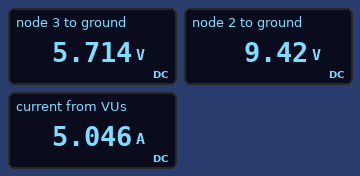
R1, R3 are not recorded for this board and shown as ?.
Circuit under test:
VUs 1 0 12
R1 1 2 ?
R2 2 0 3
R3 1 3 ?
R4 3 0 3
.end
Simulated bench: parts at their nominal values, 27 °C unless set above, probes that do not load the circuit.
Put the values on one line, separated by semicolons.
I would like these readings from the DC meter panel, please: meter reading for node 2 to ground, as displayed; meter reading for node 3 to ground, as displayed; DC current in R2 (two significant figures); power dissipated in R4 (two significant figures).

9.42 V; 5.714 V; 3.1 A; 11 W
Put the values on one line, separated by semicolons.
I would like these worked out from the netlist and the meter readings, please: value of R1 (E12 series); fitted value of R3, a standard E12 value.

0.82 Ω; 3.3 Ω
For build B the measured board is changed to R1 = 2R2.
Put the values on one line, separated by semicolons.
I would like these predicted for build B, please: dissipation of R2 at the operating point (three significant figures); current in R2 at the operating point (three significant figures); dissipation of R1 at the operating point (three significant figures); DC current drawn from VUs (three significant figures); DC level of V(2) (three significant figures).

16.0 W; 2.31 A; 11.7 W; 4.21 A; 6.92 V
